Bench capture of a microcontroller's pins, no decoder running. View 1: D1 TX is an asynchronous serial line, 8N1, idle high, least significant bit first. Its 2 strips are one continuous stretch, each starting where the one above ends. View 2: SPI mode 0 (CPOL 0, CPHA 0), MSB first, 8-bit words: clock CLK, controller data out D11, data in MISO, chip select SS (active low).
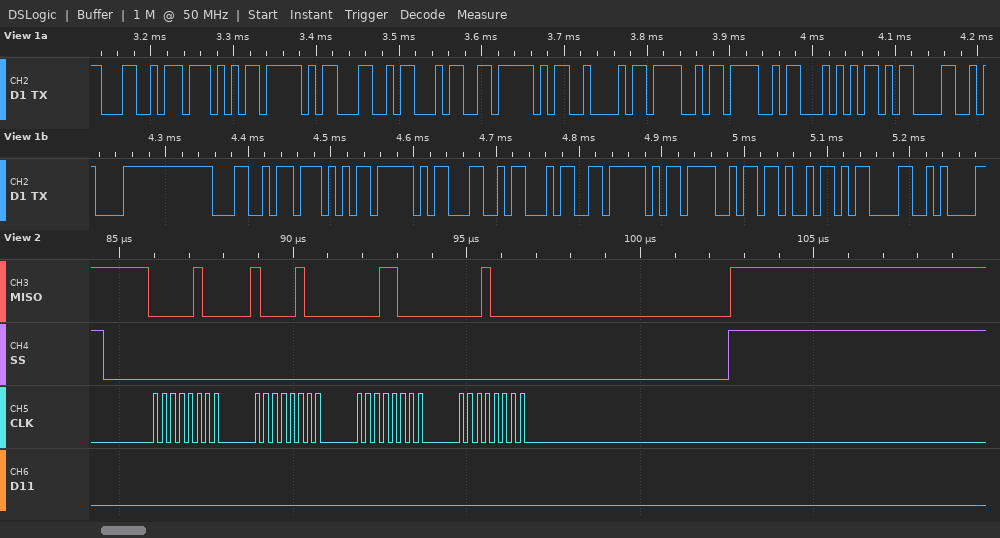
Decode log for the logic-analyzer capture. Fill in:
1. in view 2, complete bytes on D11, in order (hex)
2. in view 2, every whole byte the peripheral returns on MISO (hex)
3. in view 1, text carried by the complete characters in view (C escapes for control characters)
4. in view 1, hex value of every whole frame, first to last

00 00 00 00
04 84 18 10
"LW_L4_BOOT\r\nLW_L4_OK\r\n"
4C 57 5F 4C 34 5F 42 4F 4F 54 0D 0A 4C 57 5F 4C 34 5F 4F 4B 0D 0A
